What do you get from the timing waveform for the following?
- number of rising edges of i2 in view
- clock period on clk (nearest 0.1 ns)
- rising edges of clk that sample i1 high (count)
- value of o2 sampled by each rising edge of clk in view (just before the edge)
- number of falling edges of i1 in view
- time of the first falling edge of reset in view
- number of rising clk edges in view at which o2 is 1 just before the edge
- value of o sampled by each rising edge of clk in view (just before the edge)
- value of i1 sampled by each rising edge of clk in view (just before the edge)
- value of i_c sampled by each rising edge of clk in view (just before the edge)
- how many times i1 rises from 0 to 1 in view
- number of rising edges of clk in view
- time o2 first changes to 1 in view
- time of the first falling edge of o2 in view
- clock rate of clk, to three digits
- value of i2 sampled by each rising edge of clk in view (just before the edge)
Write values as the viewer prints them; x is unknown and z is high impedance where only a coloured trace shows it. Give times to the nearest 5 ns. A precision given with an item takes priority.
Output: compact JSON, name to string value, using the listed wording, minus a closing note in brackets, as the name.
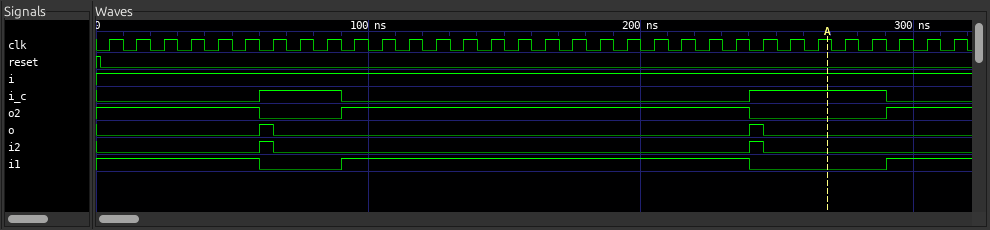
{"number of rising edges of i2 in view": "2", "clock period on clk": "10 ns", "rising edges of clk that sample i1 high": "24", "value of o2 sampled by each rising edge of clk in view": "1 1 1 1 1 1 0 0 0 1 1 1 1 1 1 1 1 1 1 1 1 1 1 1 0 0 0 0 0 1 1 1", "number of falling edges of i1 in view": "2", "time of the first falling edge of reset in view": "0 ns", "number of rising clk edges in view at which o2 is 1 just before the edge": "24", "value of o sampled by each rising edge of clk in view": "0 0 0 0 0 0 1 0 0 0 0 0 0 0 0 0 0 0 0 0 0 0 0 0 1 0 0 0 0 0 0 0", "value of i1 sampled by each rising edge of clk in view": "1 1 1 1 1 1 0 0 0 1 1 1 1 1 1 1 1 1 1 1 1 1 1 1 0 0 0 0 0 1 1 1", "value of i_c sampled by each rising edge of clk in view": "0 0 0 0 0 0 1 1 1 0 0 0 0 0 0 0 0 0 0 0 0 0 0 0 1 1 1 1 1 0 0 0", "how many times i1 rises from 0 to 1 in view": "2", "number of rising edges of clk in view": "32", "time o2 first changes to 1 in view": "90 ns", "time of the first falling edge of o2 in view": "60 ns", "clock rate of clk, to three digits": "100 MHz", "value of i2 sampled by each rising edge of clk in view": "0 0 0 0 0 0 1 0 0 0 0 0 0 0 0 0 0 0 0 0 0 0 0 0 1 0 0 0 0 0 0 0"}
